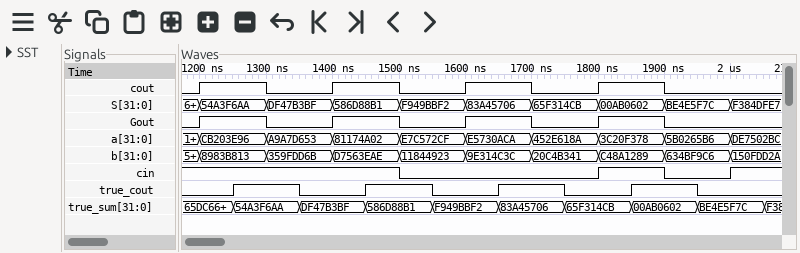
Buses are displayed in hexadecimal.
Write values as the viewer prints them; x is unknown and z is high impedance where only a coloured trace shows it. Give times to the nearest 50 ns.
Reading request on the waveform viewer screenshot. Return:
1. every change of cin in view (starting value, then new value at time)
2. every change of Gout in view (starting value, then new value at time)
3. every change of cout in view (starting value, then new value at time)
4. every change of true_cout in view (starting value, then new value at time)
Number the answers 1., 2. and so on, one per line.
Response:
1. 1, 0 at 1500 ns, 1 at 1800 ns, 0 at 1900 ns, 1 at 2000 ns
2. 0, 1 at 1200 ns, 0 at 1300 ns, 1 at 1400 ns, 0 at 1500 ns, 1 at 1600 ns, 0 at 1700 ns, 1 at 1800 ns, 0 at 1900 ns
3. 0, 1 at 1200 ns, 0 at 1300 ns, 1 at 1400 ns, 0 at 1500 ns, 1 at 1600 ns, 0 at 1700 ns, 1 at 1800 ns, 0 at 1900 ns
4. 0, 1 at 1250 ns, 0 at 1350 ns, 1 at 1450 ns, 0 at 1550 ns, 1 at 1650 ns, 0 at 1750 ns, 1 at 1850 ns, 0 at 1950 ns
